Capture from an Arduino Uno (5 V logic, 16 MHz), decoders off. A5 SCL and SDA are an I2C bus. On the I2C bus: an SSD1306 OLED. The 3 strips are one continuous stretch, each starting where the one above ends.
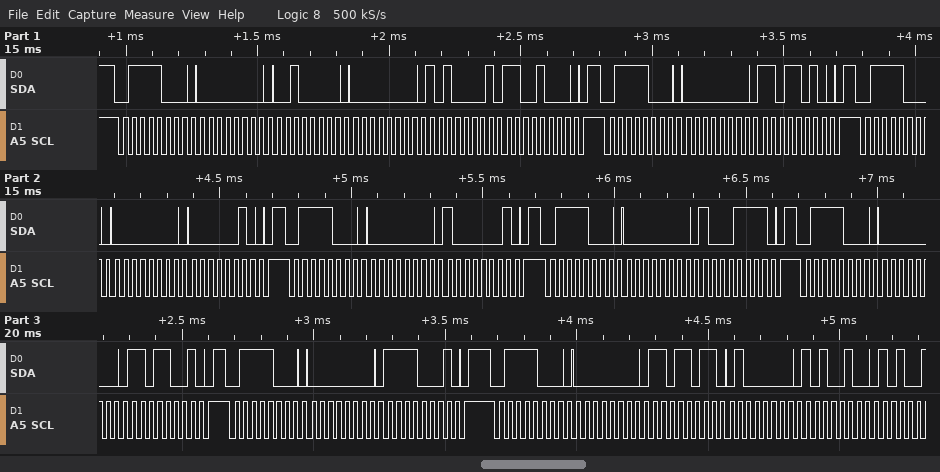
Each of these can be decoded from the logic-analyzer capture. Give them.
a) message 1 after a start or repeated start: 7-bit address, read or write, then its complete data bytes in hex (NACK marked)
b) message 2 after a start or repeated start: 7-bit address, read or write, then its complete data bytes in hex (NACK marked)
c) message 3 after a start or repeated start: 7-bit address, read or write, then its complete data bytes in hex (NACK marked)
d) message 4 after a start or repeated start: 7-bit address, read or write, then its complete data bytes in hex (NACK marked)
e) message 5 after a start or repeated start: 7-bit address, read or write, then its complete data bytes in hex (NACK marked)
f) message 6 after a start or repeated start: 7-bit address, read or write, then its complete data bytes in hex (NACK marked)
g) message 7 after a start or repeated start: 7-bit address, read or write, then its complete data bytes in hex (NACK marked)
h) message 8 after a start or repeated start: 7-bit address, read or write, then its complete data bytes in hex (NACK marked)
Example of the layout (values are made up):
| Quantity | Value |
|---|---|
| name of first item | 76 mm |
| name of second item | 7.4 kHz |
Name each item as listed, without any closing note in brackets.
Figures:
| Quantity | Value |
|---|---|
| message 1 after a start or repeated start: 7-bit address, read or write, then its complete data bytes in hex | 0x3C write: 00 20 00 A1 C8 |
| message 2 after a start or repeated start: 7-bit address, read or write, then its complete data bytes in hex | 0x3C write: 00 DA |
| message 3 after a start or repeated start: 7-bit address, read or write, then its complete data bytes in hex | 0x3C write: 00 02 |
| message 4 after a start or repeated start: 7-bit address, read or write, then its complete data bytes in hex | 0x3C write: 00 81 |
| message 5 after a start or repeated start: 7-bit address, read or write, then its complete data bytes in hex | 0x3C write: 00 8F |
| message 6 after a start or repeated start: 7-bit address, read or write, then its complete data bytes in hex | 0x3C write: 00 D9 |
| message 7 after a start or repeated start: 7-bit address, read or write, then its complete data bytes in hex | 0x3C write: 00 F1 |
| message 8 after a start or repeated start: 7-bit address, read or write, then its complete data bytes in hex | 0x3C write: 00 DB 40 A4 |
